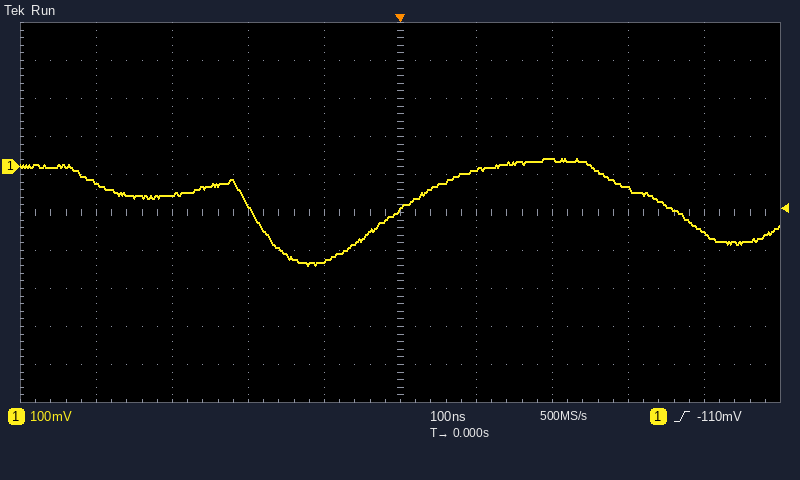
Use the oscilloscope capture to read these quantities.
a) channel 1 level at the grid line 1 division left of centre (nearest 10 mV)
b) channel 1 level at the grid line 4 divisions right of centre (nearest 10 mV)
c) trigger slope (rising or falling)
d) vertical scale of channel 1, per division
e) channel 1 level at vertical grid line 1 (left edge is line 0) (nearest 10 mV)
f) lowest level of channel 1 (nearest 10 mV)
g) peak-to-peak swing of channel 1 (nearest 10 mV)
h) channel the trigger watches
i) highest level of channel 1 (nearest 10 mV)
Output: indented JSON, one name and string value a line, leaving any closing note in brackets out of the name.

{
  "channel 1 level at the grid line 1 division left of centre": "-250 mV",
  "channel 1 level at the grid line 4 divisions right of centre": "-170 mV",
  "trigger slope": "rising",
  "vertical scale of channel 1, per division": "100 mV",
  "channel 1 level at vertical grid line 1 (left edge is line 0)": "-40 mV",
  "lowest level of channel 1": "-260 mV",
  "peak-to-peak swing of channel 1": "280 mV",
  "channel the trigger watches": "channel 1",
  "highest level of channel 1": "20 mV"
}
